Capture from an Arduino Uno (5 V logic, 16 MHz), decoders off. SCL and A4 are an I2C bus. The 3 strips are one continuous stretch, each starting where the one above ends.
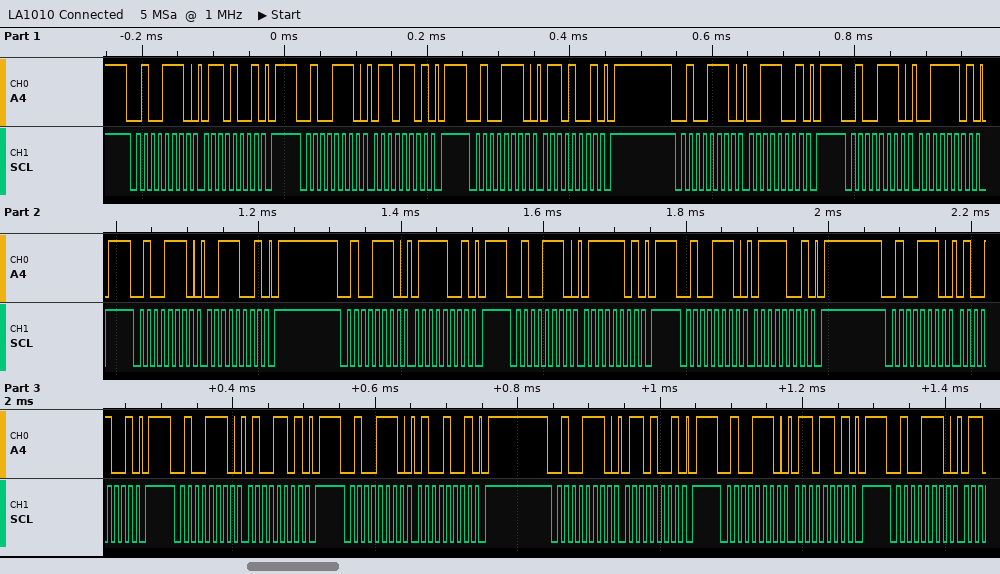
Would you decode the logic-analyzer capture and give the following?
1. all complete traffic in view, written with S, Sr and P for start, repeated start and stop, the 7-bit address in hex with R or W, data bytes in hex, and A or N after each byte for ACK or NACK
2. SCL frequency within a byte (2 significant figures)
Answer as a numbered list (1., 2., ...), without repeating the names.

1. S 27W A 69 A P S 27W A 6D A P S 27W A 69 A P S 27W A 39 A P S 27W A 3D A P S 27W A 39 A P S 27W A 79 A P S 27W A 7D A P S 27W A 79 A P S 27W A 49 A P S 27W A 4D A P S 27W A 49 A P S 27W A 69 A P S 27W A 6D A P S 27W A
2. 100 kHz
